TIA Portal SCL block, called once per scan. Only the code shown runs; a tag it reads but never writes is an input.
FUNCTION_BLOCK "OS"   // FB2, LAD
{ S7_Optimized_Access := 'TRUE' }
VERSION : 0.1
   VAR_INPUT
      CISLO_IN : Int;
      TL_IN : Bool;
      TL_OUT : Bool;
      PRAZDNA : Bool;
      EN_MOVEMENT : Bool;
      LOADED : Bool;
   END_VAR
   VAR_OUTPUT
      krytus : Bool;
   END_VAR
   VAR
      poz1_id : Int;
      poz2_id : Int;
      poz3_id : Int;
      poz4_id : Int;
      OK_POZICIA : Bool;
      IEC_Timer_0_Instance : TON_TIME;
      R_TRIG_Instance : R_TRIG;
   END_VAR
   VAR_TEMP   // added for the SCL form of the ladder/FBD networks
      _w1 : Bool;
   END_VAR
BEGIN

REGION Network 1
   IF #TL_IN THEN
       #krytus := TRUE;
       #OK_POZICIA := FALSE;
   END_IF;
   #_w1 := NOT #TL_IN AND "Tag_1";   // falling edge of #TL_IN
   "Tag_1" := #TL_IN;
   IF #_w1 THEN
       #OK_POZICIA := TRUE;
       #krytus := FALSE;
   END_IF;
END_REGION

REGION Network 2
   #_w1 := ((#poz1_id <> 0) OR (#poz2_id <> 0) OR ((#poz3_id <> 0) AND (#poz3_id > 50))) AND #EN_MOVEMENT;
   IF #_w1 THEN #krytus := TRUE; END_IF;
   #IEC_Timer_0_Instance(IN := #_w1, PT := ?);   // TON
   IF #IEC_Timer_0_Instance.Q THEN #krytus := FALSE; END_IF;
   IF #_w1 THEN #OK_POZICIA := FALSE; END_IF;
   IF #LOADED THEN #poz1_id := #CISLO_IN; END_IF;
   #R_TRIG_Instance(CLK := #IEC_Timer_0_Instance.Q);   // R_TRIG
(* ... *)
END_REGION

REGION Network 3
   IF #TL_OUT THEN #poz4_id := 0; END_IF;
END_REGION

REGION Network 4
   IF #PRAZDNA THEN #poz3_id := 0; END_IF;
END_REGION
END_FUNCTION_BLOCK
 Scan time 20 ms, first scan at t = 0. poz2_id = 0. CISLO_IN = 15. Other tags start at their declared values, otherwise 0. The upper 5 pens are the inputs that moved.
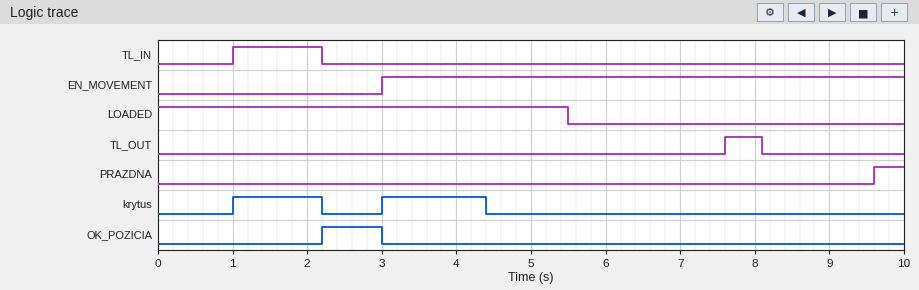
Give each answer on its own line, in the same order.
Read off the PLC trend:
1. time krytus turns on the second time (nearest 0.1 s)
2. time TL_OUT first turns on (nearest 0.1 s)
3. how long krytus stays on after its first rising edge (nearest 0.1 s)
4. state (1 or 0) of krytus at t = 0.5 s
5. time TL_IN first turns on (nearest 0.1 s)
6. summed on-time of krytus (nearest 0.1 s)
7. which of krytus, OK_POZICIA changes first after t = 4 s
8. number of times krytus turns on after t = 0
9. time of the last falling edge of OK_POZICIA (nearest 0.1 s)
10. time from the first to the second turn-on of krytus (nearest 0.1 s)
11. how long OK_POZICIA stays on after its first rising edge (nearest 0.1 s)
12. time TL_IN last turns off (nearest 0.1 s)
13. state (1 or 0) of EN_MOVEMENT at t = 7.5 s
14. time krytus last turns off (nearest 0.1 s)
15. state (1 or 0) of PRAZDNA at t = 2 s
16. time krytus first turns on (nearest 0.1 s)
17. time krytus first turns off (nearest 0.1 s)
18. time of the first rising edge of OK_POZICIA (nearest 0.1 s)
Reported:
3.0 s
7.6 s
1.2 s
0
1.0 s
2.6 s
krytus
2
3.0 s
2.0 s
0.8 s
2.2 s
1
4.4 s
0
1.0 s
2.2 s
2.2 s
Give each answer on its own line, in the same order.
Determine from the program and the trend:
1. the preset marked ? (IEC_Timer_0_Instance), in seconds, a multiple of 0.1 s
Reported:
1.4 s
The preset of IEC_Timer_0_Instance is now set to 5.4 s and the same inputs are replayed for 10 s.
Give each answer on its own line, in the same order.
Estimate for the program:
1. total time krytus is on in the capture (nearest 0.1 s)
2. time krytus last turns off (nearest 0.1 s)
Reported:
6.6 s
8.4 s
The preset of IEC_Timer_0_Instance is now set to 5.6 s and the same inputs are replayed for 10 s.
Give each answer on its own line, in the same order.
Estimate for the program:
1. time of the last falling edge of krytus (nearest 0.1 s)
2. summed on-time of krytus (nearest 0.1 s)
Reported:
8.6 s
6.8 s
